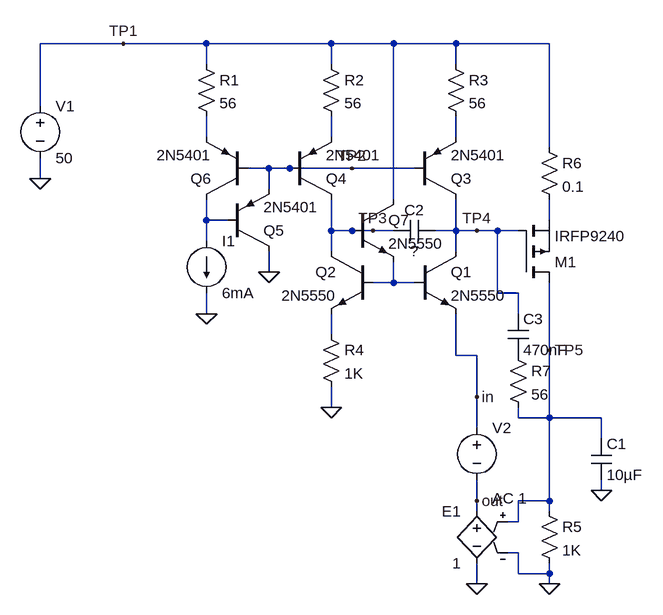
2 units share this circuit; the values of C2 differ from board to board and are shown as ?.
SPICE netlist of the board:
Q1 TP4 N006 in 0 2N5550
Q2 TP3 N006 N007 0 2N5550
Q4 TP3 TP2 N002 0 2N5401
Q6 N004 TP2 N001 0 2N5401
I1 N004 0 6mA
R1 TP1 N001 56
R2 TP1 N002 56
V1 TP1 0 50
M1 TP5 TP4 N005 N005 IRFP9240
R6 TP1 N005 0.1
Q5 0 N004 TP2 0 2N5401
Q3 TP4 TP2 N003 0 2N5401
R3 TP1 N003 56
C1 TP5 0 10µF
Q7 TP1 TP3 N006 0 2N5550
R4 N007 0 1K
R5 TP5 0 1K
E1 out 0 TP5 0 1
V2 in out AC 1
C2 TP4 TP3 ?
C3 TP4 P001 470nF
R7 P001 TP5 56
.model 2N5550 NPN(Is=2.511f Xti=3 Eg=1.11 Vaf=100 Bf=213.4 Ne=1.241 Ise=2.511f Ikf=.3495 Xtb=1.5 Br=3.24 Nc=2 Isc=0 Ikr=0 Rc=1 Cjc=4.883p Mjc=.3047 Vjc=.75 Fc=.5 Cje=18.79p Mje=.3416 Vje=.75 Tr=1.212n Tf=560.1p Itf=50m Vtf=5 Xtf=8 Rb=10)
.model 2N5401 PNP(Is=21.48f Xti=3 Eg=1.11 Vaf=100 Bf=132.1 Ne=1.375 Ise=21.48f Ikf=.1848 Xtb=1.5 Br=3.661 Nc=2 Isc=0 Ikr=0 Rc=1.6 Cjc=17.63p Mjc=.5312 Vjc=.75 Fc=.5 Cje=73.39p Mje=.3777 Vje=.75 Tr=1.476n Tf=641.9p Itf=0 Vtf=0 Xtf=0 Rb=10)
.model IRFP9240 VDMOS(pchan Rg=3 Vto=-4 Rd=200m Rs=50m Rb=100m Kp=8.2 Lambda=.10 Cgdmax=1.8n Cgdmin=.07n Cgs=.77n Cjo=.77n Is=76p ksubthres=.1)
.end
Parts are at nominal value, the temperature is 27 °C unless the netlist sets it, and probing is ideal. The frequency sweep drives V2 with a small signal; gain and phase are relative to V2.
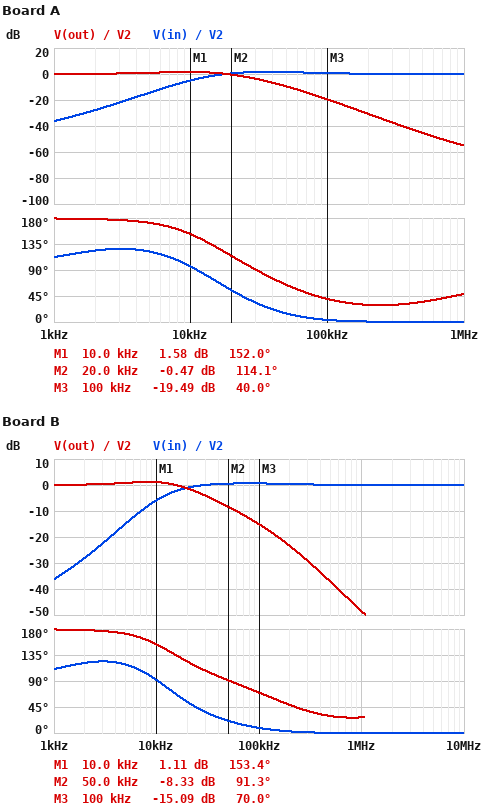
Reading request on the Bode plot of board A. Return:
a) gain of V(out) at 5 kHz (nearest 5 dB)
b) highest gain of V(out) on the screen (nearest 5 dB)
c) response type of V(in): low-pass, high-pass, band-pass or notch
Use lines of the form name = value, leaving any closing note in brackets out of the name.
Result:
gain of V(out) at 5 kHz = 0 dB
highest gain of V(out) on the screen = 0 dB
response type of V(in): low-pass, high-pass, band-pass or notch = high-pass
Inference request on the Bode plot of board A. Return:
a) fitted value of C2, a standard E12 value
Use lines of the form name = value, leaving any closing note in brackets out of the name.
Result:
fitted value of C2, a standard E12 value = 180 pF
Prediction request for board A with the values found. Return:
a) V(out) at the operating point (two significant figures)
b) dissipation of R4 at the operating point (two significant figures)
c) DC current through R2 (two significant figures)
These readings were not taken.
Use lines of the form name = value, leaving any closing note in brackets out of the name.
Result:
V(out) at the operating point = 6.2 V
dissipation of R4 at the operating point = 39 mW
DC current through R2 = 6.2 mA
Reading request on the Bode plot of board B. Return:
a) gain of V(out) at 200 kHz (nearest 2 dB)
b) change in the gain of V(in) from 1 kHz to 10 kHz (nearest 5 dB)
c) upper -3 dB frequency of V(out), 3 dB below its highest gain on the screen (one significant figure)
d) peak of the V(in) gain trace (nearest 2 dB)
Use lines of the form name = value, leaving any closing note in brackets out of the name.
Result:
gain of V(out) at 200 kHz = -24 dB
change in the gain of V(in) from 1 kHz to 10 kHz = 30 dB
upper -3 dB frequency of V(out), 3 dB below its highest gain on the screen = 20 kHz
peak of the V(in) gain trace = 0 dB
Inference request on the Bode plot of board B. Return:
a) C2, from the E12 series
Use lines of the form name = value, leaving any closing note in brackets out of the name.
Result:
C2, from the E12 series = 56 pF
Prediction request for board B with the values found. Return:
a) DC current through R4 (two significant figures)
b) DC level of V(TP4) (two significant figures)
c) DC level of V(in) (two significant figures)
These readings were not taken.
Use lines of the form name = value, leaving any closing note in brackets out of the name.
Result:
DC current through R4 = 6.2 mA
DC level of V(TP4) = 46 V
DC level of V(in) = 6.2 V
